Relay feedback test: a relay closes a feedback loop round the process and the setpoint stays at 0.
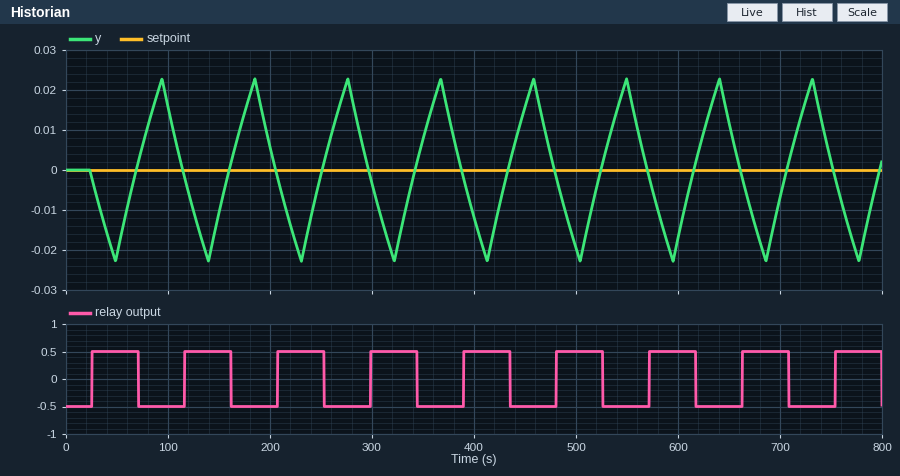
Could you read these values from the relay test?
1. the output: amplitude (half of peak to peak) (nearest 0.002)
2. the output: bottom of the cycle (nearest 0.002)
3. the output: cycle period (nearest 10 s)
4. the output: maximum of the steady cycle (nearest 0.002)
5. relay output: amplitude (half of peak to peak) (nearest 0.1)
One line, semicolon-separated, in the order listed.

0.022; -0.022; 90 s; 0.022; 0.5
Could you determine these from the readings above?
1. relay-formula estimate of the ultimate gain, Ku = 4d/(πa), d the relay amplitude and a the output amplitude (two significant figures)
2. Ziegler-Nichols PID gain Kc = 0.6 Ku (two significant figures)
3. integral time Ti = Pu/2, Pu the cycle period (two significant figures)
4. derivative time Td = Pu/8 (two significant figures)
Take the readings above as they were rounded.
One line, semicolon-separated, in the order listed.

29; 17; 45 s; 11 s
